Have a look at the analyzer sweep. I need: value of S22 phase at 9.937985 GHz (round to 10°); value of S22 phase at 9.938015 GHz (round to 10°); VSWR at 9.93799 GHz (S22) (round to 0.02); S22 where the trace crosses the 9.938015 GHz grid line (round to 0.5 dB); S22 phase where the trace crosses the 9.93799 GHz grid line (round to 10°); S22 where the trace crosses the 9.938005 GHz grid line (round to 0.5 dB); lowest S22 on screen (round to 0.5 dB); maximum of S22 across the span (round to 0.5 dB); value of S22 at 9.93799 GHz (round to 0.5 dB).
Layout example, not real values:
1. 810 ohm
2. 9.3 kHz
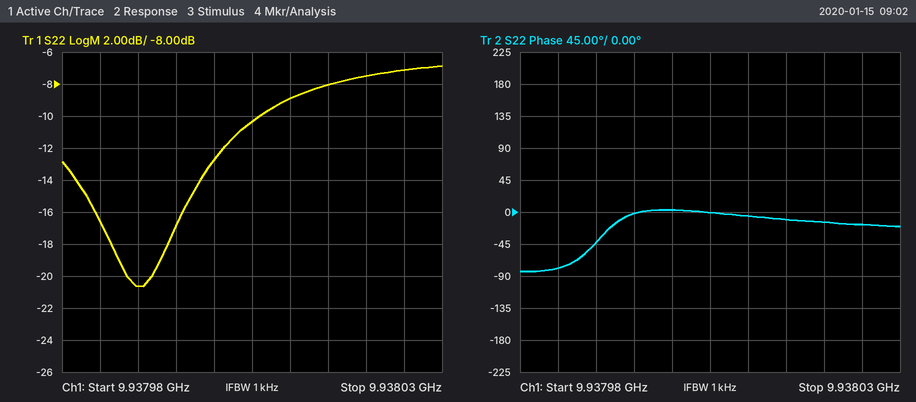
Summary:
1. -80°
2. -10°
3. 1.20
4. -8.0 dB
5. -40°
6. -10.5 dB
7. -20.5 dB
8. -7.0 dB
9. -20.5 dB
